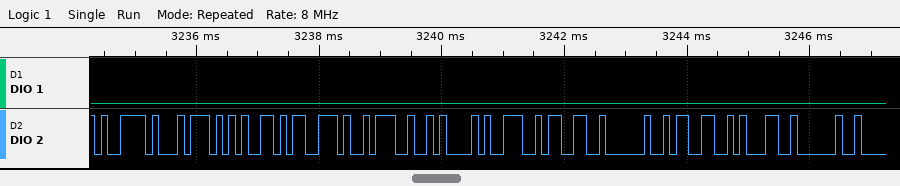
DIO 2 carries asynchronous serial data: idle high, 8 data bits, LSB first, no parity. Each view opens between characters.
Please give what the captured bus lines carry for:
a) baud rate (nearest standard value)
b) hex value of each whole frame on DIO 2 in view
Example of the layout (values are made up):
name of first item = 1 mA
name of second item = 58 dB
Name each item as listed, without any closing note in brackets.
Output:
baud rate = 9600 baud
hex value of each whole frame on DIO 2 in view = 79, 74, 65, 73, 3A, 0A, 39, 33, 20, 33, 31, 20
